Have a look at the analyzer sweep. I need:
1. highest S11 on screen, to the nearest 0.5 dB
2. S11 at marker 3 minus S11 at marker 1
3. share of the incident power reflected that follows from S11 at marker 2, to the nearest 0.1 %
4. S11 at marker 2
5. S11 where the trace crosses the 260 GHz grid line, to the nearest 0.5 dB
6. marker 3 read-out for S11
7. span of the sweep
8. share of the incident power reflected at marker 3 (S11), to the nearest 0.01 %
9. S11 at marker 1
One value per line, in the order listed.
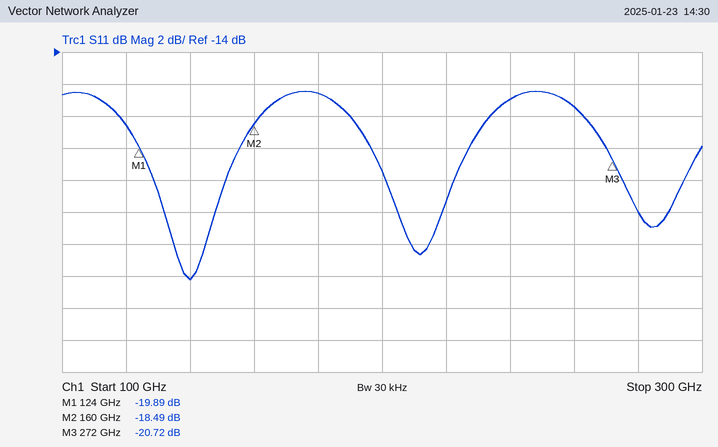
-16.5 dB
-0.83 dB
1.4 %
-18.49 dB
-17.5 dB
-20.72 dB
200 GHz
0.85 %
-19.89 dB
